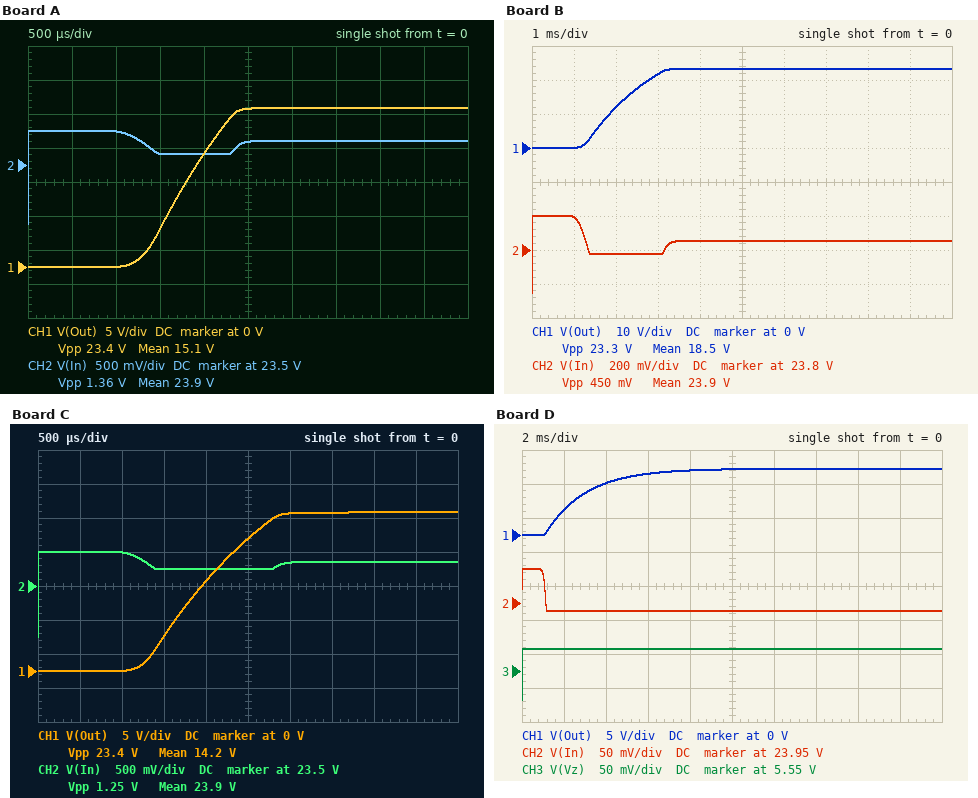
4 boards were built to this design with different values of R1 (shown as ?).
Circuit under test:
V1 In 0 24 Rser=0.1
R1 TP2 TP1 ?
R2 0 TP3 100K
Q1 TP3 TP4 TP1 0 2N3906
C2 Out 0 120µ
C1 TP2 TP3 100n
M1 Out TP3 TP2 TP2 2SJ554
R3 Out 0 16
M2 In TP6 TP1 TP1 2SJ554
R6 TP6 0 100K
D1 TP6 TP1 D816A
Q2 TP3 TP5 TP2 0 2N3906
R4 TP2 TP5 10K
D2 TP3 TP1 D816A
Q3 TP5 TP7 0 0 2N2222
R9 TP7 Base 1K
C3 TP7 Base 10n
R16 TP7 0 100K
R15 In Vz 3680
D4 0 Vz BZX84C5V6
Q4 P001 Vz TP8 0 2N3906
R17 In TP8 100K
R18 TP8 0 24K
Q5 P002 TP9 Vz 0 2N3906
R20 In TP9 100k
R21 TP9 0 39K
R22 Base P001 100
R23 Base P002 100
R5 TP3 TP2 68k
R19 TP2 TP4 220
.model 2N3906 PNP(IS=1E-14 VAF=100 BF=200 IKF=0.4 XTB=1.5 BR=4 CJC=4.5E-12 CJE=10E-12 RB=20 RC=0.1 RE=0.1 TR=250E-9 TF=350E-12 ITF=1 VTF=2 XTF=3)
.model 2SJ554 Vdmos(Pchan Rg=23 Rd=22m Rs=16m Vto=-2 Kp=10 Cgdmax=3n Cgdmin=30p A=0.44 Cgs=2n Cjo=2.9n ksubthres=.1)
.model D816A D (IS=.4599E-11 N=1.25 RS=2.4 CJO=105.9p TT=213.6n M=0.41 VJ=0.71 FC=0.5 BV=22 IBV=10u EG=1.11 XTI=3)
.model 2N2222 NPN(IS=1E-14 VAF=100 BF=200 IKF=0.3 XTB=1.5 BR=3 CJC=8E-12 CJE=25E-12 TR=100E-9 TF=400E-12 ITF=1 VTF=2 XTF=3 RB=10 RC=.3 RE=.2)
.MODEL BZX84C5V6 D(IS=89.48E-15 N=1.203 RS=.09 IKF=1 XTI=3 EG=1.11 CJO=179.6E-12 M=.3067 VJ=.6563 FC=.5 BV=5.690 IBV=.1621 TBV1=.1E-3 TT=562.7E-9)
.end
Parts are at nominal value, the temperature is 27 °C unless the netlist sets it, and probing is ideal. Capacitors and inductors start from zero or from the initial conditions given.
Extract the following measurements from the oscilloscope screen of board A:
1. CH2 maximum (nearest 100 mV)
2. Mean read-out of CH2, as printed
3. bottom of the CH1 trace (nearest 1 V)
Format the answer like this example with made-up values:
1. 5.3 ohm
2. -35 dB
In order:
1. 24.0 V
2. 23.9 V
3. 0 V
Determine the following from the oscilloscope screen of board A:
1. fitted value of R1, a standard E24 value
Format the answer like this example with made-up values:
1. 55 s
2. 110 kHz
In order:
1. 0.18 Ω
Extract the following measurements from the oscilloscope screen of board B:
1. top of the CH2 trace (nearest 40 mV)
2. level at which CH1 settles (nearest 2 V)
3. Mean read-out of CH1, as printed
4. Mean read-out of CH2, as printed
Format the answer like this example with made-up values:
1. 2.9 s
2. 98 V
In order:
1. 24.00 V
2. 24 V
3. 18.5 V
4. 23.9 V
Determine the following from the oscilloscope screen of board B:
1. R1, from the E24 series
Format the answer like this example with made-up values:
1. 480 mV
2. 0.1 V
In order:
1. 0.27 Ω
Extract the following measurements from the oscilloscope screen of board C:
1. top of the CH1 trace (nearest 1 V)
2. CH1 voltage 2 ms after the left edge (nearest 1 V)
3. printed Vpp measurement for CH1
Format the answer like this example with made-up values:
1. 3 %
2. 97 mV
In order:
1. 23 V
2. 13 V
3. 23.4 V
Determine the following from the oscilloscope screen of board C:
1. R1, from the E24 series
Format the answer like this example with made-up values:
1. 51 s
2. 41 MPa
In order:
1. 0.24 Ω
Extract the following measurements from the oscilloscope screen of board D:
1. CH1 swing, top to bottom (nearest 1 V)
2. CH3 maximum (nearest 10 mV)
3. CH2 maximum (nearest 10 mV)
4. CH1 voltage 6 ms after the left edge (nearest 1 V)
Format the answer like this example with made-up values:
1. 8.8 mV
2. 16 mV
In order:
1. 10 V
2. 5.58 V
3. 24.00 V
4. 9 V
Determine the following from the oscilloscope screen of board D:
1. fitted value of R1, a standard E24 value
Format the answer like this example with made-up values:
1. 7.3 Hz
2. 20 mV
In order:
1. 1 Ω
